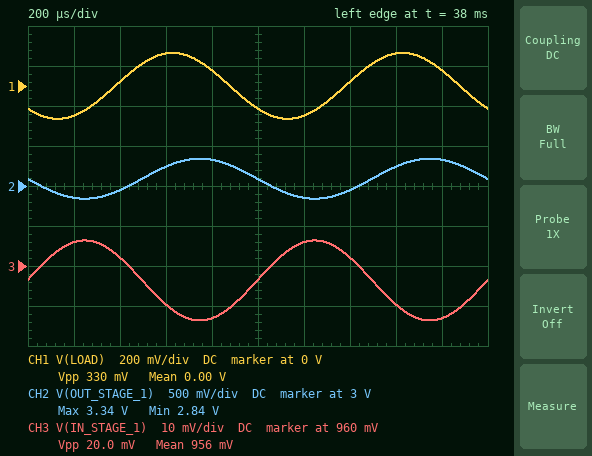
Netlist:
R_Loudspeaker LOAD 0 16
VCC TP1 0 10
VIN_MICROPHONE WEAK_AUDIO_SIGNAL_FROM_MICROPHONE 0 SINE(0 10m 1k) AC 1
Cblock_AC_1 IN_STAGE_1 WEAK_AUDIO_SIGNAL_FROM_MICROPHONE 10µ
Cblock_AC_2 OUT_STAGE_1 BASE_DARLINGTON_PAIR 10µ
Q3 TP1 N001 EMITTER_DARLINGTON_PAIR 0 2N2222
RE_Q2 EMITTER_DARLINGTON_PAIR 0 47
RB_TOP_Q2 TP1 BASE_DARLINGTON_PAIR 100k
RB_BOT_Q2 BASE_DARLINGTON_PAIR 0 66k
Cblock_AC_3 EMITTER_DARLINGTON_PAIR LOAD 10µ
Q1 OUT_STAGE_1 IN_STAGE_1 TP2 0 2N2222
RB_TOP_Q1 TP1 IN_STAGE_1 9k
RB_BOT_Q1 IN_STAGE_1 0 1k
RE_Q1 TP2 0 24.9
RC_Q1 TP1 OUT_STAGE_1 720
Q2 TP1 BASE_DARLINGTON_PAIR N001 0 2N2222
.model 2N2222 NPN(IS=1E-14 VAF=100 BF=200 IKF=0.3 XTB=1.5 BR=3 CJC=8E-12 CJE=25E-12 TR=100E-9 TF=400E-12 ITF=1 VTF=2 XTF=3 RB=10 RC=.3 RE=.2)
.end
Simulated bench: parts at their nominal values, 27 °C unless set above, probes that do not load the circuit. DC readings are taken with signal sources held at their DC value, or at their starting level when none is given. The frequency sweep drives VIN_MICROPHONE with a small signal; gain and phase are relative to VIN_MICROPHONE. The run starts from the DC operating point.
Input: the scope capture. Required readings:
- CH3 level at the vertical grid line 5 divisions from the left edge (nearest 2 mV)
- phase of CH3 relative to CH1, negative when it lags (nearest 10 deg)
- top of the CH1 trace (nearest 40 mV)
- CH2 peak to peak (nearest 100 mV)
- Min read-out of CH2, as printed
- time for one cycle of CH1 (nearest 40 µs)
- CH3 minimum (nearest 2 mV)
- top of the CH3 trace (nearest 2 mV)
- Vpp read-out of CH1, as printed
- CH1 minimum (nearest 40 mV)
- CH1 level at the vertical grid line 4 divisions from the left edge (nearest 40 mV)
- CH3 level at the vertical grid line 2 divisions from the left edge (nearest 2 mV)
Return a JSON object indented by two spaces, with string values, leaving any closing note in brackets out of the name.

{
  "CH3 level at the vertical grid line 5 divisions from the left edge": "956 mV",
  "phase of CH3 relative to CH1, negative when it lags": "140 deg",
  "top of the CH1 trace": "160 mV",
  "CH2 peak to peak": "500 mV",
  "Min read-out of CH2, as printed": "2.84 V",
  "time for one cycle of CH1": "1.00 ms",
  "CH3 minimum": "946 mV",
  "top of the CH3 trace": "966 mV",
  "Vpp read-out of CH1, as printed": "330 mV",
  "CH1 minimum": "-160 mV",
  "CH1 level at the vertical grid line 4 divisions from the left edge": "80 mV",
  "CH3 level at the vertical grid line 2 divisions from the left edge": "962 mV"
}
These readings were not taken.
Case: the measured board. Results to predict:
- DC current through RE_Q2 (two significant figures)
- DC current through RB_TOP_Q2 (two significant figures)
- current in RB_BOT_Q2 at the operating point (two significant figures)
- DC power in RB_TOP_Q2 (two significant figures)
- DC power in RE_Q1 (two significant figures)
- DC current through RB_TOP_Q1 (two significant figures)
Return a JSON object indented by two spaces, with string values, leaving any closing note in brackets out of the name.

{
  "DC current through RE_Q2": "54 mA",
  "DC current through RB_TOP_Q2": "61 µA",
  "current in RB_BOT_Q2 at the operating point": "59 µA",
  "DC power in RB_TOP_Q2": "370 µW",
  "DC power in RE_Q1": "2.3 mW",
  "DC current through RB_TOP_Q1": "1.0 mA"
}
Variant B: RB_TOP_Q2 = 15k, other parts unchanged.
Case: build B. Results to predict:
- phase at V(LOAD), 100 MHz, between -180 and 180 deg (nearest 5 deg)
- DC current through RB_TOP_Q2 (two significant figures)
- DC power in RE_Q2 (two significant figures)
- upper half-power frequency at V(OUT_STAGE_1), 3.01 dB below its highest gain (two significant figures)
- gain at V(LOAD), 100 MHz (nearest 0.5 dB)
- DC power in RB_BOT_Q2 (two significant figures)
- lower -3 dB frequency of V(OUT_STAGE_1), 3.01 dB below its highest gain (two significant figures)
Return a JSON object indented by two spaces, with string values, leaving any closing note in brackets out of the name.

{
  "phase at V(LOAD), 100 MHz, between -180 and 180 deg": "40 deg",
  "DC current through RB_TOP_Q2": "130 µA",
  "DC power in RE_Q2": "930 mW",
  "upper half-power frequency at V(OUT_STAGE_1), 3.01 dB below its highest gain": "19 MHz",
  "gain at V(LOAD), 100 MHz": "1.0 dB",
  "DC power in RB_BOT_Q2": "990 µW",
  "lower -3 dB frequency of V(OUT_STAGE_1), 3.01 dB below its highest gain": "21 Hz"
}
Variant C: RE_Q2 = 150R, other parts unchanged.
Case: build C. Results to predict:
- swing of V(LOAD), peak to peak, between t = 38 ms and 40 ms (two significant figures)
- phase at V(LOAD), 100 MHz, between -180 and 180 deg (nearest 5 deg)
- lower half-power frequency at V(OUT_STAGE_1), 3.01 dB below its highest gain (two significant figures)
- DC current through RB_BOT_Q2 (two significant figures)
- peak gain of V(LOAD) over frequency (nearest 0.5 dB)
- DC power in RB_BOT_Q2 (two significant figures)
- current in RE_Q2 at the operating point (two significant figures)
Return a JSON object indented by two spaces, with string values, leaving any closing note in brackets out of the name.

{
  "swing of V(LOAD), peak to peak, between t = 38 ms and 40 ms": "310 mV",
  "phase at V(LOAD), 100 MHz, between -180 and 180 deg": "70 deg",
  "lower half-power frequency at V(OUT_STAGE_1), 3.01 dB below its highest gain": "23 Hz",
  "DC current through RB_BOT_Q2": "60 µA",
  "peak gain of V(LOAD) over frequency": "26.0 dB",
  "DC power in RB_BOT_Q2": "240 µW",
  "current in RE_Q2 at the operating point": "18 mA"
}
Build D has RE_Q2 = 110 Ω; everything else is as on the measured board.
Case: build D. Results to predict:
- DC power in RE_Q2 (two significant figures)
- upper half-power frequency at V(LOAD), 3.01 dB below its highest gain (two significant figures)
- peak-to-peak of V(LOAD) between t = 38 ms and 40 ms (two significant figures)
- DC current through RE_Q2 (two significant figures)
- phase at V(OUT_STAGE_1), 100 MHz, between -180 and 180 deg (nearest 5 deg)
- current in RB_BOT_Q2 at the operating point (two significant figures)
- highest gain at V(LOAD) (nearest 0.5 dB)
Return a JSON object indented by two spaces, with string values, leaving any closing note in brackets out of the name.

{
  "DC power in RE_Q2": "62 mW",
  "upper half-power frequency at V(LOAD), 3.01 dB below its highest gain": "10 MHz",
  "peak-to-peak of V(LOAD) between t = 38 ms and 40 ms": "320 mV",
  "DC current through RE_Q2": "24 mA",
  "phase at V(OUT_STAGE_1), 100 MHz, between -180 and 180 deg": "80 deg",
  "current in RB_BOT_Q2 at the operating point": "60 µA",
  "highest gain at V(LOAD)": "26.5 dB"
}
